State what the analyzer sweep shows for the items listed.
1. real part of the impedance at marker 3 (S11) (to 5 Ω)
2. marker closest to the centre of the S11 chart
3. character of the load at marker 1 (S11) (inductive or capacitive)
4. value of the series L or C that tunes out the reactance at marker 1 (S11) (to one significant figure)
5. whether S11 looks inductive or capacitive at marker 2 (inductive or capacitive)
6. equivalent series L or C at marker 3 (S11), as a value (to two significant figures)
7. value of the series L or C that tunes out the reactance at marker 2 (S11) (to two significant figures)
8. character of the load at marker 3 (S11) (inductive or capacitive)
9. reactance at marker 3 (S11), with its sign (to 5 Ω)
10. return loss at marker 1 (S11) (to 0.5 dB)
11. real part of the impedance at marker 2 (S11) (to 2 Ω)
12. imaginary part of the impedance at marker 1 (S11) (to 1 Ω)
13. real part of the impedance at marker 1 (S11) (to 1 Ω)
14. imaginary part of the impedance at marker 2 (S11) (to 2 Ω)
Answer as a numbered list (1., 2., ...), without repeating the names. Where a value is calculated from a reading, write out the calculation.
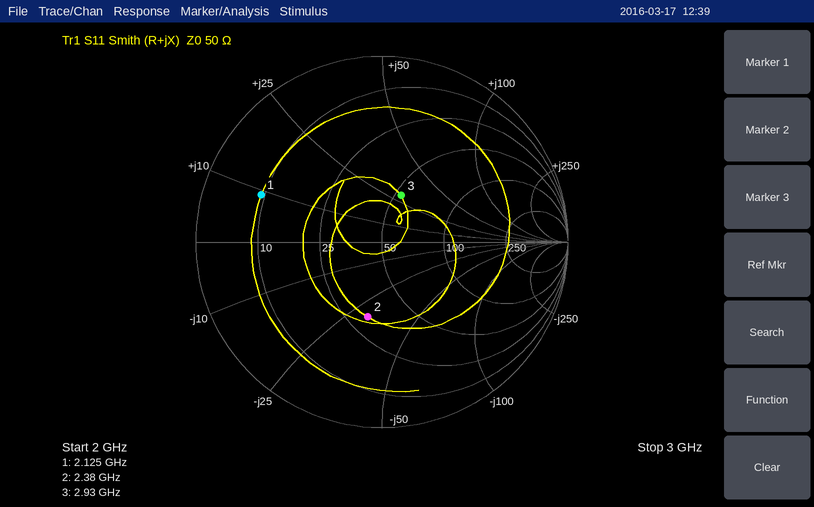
1. 55 Ω
2. marker 3
3. inductive
4. C = 1/(2π × 2.125 GHz × 9 Ω) ≈ 8 pF
5. capacitive
6. L = 30 Ω/(2π × 2.93 GHz) ≈ 1.6 nH
7. L = 30 Ω/(2π × 2.38 GHz) ≈ 2.0 nH
8. inductive
9. +30 Ω
10. 3.0 dB
11. 32 Ω
12. +9 Ω
13. 9 Ω
14. -30 Ω
